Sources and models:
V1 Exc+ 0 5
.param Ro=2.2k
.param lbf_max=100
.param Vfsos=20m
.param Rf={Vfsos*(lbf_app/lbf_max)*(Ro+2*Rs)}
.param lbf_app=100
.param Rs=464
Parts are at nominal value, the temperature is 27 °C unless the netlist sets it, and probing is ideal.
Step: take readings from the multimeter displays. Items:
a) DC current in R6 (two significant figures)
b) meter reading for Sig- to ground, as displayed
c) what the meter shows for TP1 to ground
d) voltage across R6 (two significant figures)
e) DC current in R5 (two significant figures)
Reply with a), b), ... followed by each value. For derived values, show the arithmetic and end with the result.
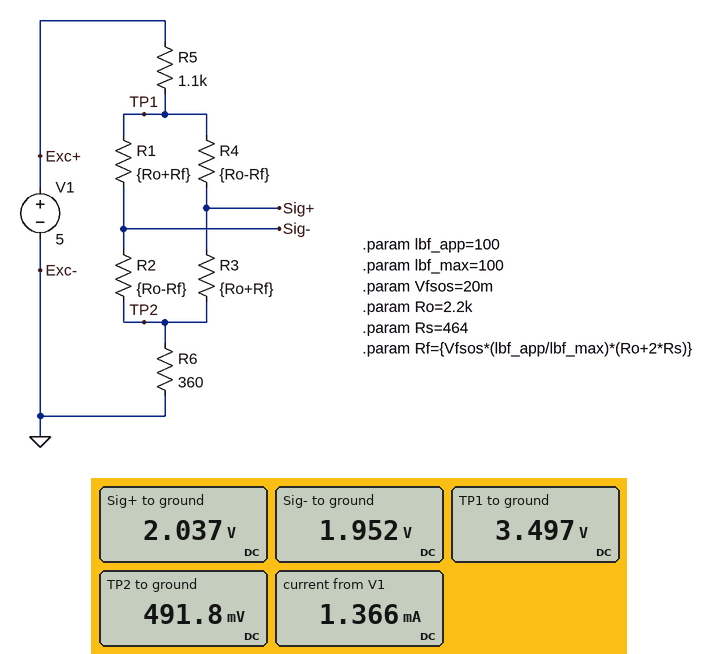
a) (491.8 mV) / 360 Ω = 1.4 mA
b) 1.952 V
c) 3.497 V
d) 491.8 mV = 490 mV
e) (5 V - 3.497 V) / 1.1 kΩ = 1.4 mA
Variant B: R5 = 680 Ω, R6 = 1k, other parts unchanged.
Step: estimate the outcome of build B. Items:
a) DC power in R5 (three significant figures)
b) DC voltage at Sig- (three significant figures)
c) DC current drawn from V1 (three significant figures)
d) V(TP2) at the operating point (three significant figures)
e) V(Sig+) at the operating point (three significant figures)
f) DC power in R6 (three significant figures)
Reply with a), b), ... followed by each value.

a) 1.13 mW
b) 2.67 V
c) 1.29 mA
d) 1.29 V
e) 2.75 V
f) 1.66 mW
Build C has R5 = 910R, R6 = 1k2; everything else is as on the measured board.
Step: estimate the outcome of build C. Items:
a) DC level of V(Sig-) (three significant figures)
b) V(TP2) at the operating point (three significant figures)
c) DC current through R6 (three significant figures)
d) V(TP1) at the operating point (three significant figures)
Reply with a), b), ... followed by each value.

a) 2.63 V
b) 1.39 V
c) 1.16 mA
d) 3.94 V
